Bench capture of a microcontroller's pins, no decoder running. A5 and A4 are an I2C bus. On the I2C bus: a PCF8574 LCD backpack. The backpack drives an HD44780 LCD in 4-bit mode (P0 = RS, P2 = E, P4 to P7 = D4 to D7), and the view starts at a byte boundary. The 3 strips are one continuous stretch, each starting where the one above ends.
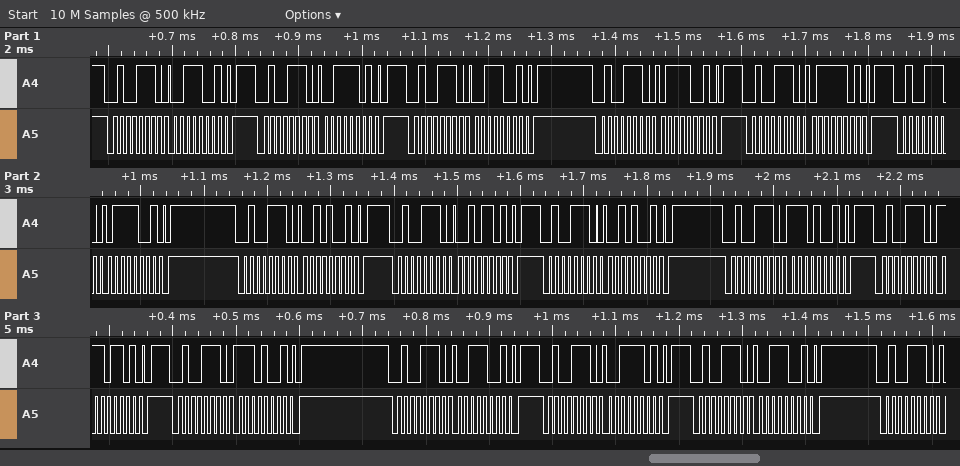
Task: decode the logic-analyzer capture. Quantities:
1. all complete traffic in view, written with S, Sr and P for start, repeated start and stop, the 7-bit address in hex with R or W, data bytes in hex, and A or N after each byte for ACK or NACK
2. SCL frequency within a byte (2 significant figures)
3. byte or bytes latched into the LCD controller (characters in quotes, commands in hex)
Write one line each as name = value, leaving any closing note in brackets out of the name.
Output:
all complete traffic in view, written with S, Sr and P for start, repeated start and stop, the 7-bit address in hex with R or W, data bytes in hex, and A or N after each byte for ACK or NACK = S 27W A 39 A P S 27W A 3D A P S 27W A 39 A P S 27W A 79 A P S 27W A 7D A P S 27W A 79 A P S 27W A 29 A P S 27W A 2D A P S 27W A 29 A P S 27W A E9 A P S 27W A ED A P S 27W A E9 A P S 27W A 39 A P S 27W A 3D A P S 27W A 39 A P S 27W A
SCL frequency within a byte = 100 kHz
byte or bytes latched into the LCD controller = '7' '.'
